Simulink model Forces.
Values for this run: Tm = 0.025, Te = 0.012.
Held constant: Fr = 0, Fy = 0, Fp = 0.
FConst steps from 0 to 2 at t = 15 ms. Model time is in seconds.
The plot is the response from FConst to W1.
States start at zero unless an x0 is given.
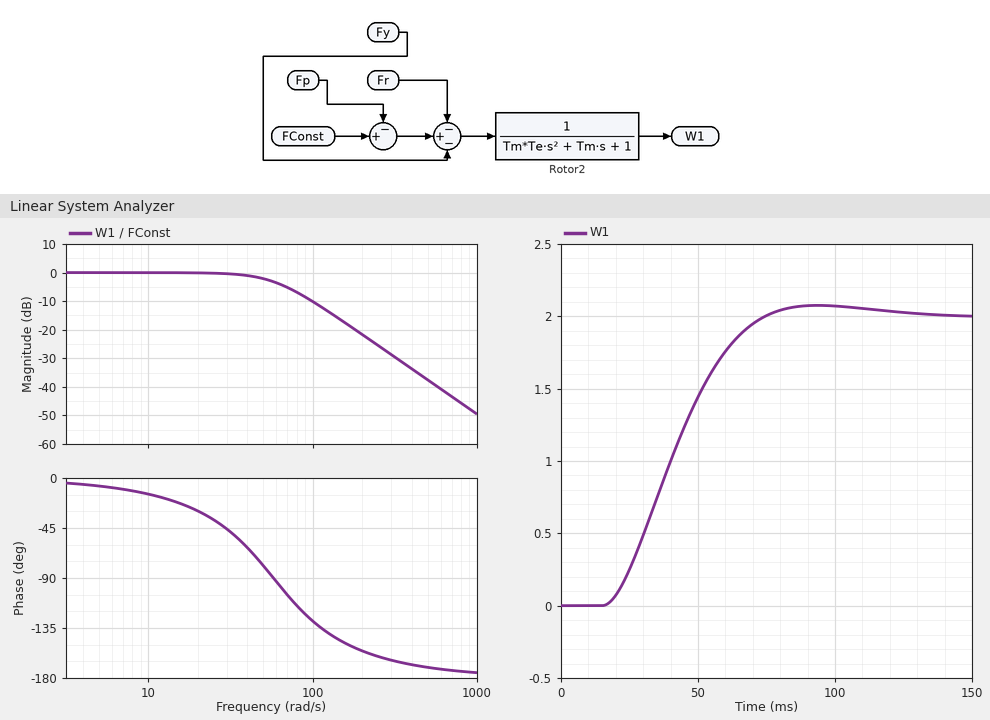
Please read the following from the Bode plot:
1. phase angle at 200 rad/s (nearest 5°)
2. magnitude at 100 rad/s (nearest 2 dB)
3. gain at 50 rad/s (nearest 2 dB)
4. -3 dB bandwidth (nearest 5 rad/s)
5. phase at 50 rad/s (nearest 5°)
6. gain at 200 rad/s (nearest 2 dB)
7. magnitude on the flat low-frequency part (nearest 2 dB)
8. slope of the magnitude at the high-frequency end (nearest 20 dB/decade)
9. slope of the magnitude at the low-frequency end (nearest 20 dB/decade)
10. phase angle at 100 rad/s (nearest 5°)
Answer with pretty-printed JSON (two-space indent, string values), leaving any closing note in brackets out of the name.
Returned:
{
  "phase angle at 200 rad/s": "-155°",
  "magnitude at 100 rad/s": "-10 dB",
  "gain at 50 rad/s": "-2 dB",
  "-3 dB bandwidth": "55 rad/s",
  "phase at 50 rad/s": "-80°",
  "gain at 200 rad/s": "-22 dB",
  "magnitude on the flat low-frequency part": "0 dB",
  "slope of the magnitude at the high-frequency end": "-40 dB/decade",
  "slope of the magnitude at the low-frequency end": "0 dB/decade",
  "phase angle at 100 rad/s": "-130°"
}
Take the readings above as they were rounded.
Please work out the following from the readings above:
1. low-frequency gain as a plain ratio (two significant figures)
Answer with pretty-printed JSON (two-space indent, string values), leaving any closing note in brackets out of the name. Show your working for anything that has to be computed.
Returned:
{
  "low-frequency gain as a plain ratio": "10^(0 / 20) = 1.0"
}
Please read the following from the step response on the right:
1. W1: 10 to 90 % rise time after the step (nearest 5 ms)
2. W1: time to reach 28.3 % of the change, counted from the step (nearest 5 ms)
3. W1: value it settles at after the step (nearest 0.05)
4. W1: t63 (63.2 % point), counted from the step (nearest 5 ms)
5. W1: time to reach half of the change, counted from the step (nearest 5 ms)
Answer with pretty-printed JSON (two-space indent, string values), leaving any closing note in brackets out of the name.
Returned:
{
  "W1: 10 to 90 % rise time after the step": "40 ms",
  "W1: time to reach 28.3 % of the change, counted from the step": "15 ms",
  "W1: value it settles at after the step": "2.00",
  "W1: t63 (63.2 % point), counted from the step": "30 ms",
  "W1: time to reach half of the change, counted from the step": "25 ms"
}
